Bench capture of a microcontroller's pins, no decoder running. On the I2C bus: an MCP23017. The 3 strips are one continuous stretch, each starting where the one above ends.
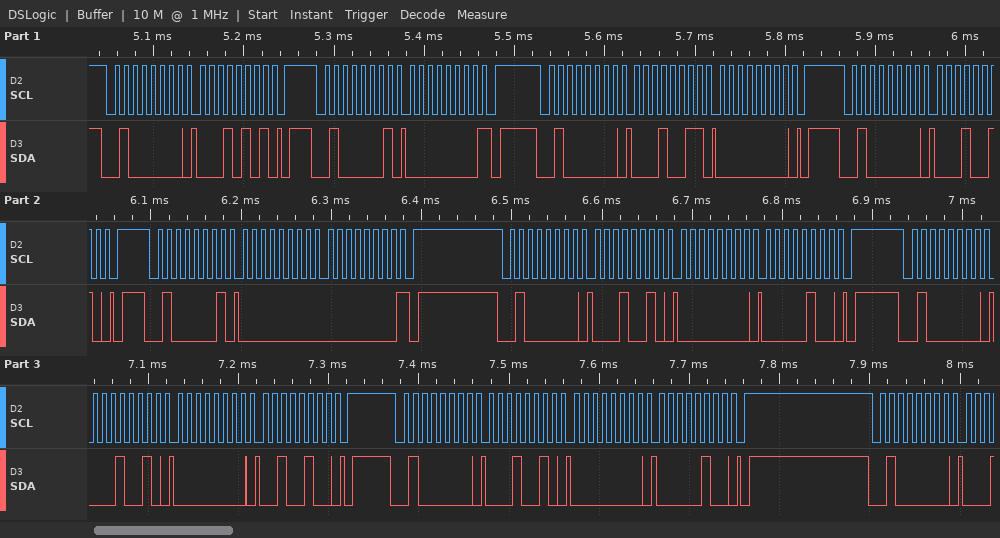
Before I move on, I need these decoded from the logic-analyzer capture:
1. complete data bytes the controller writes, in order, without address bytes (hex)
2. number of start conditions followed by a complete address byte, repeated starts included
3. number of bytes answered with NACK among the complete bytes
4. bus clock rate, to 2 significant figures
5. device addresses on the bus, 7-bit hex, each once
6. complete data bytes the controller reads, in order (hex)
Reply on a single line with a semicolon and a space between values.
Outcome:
15 13 00 12 12 00 04 12 00 24 12 00 04; 9; 2; 100 kHz; 0x20; 00 00 00
